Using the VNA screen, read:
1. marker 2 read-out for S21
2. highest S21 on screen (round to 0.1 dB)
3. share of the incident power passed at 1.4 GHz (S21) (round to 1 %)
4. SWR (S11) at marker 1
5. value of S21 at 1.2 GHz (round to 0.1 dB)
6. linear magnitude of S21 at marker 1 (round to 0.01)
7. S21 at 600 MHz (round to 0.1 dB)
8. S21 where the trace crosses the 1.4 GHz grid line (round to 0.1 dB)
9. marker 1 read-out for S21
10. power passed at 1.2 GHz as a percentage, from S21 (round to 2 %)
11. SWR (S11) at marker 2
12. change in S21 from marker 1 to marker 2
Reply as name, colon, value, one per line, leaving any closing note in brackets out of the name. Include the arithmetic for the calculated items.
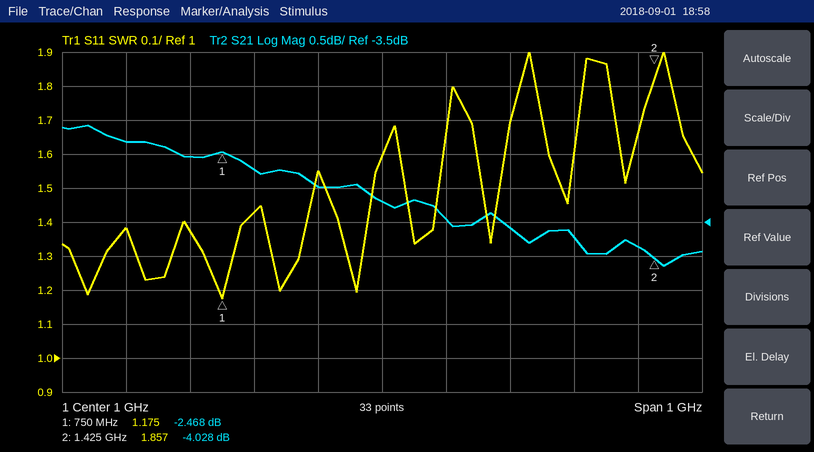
marker 2 read-out for S21: -4.028 dB
highest S21 on screen: -2.1 dB
share of the incident power passed at 1.4 GHz (S21): 10^(-3.9/10) ≈ 41 %
SWR (S11) at marker 1: 1.175
value of S21 at 1.2 GHz: -3.6 dB
linear magnitude of S21 at marker 1: 10^(-2.468/20) ≈ 0.75
S21 at 600 MHz: -2.3 dB
S21 where the trace crosses the 1.4 GHz grid line: -3.9 dB
marker 1 read-out for S21: -2.468 dB
power passed at 1.2 GHz as a percentage, from S21: 10^(-3.6/10) ≈ 44 %
SWR (S11) at marker 2: 1.857
change in S21 from marker 1 to marker 2: -4.028 − (-2.468) = -1.560 dB
